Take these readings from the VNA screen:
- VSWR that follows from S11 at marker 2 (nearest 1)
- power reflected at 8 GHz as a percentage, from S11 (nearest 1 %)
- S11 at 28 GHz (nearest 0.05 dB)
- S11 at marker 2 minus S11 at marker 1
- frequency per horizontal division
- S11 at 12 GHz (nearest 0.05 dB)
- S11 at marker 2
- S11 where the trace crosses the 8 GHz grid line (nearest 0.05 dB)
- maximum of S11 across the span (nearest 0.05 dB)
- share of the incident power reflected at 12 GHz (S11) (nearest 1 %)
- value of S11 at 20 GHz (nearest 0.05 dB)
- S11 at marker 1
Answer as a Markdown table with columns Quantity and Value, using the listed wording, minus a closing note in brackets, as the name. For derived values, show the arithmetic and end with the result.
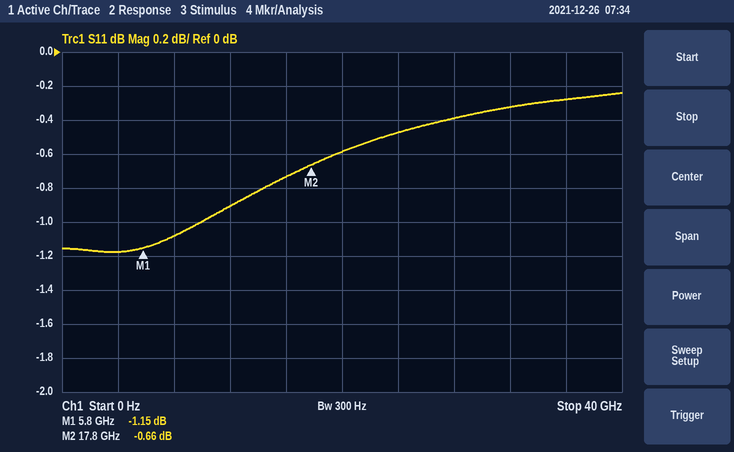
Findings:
| Quantity | Value |
|---|---|
| VSWR that follows from S11 at marker 2 | (1 + 0.9268)/(1 − 0.9268) ≈ 26 |
| power reflected at 8 GHz as a percentage, from S11 | 10^(-1.1/10) ≈ 78 % |
| S11 at 28 GHz | -0.40 dB |
| S11 at marker 2 minus S11 at marker 1 | -0.66 − (-1.15) = 0.49 dB |
| frequency per horizontal division | 4 GHz |
| S11 at 12 GHz | -0.90 dB |
| S11 at marker 2 | -0.66 dB |
| S11 where the trace crosses the 8 GHz grid line | -1.10 dB |
| maximum of S11 across the span | -0.25 dB |
| share of the incident power reflected at 12 GHz (S11) | 10^(-0.9/10) ≈ 81 % |
| value of S11 at 20 GHz | -0.60 dB |
| S11 at marker 1 | -1.15 dB |
